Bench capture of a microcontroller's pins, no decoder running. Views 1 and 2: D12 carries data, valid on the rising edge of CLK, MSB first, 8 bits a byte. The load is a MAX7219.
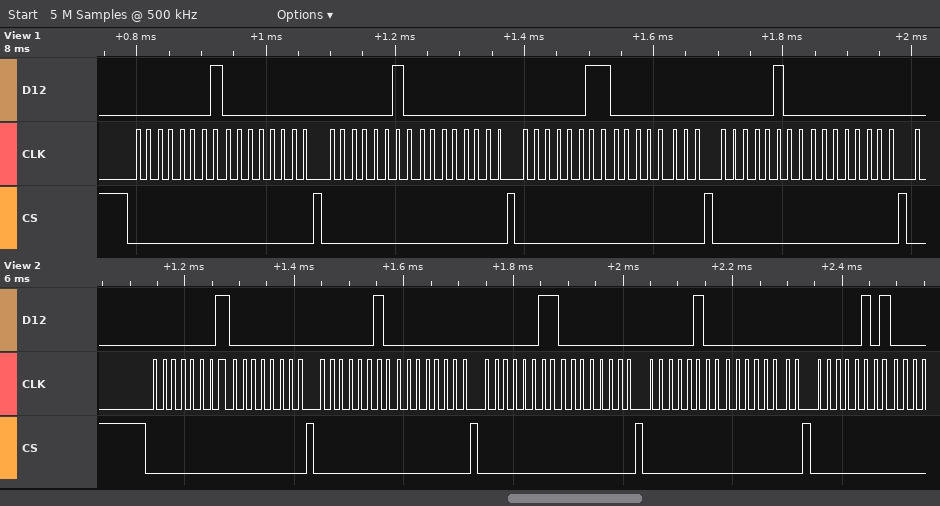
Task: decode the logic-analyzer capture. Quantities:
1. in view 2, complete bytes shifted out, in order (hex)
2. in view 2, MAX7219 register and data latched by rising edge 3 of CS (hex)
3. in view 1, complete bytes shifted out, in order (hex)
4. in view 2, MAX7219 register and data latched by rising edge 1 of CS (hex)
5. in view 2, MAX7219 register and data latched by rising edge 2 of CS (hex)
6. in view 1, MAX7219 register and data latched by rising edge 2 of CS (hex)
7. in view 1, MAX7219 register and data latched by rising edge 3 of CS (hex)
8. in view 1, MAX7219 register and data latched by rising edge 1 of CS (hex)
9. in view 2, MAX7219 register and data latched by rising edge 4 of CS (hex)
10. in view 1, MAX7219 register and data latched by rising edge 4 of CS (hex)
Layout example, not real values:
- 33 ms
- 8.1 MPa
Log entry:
- 01 00 02 00 03 00 04 00 05
- register 0x3, data 0x00
- 01 00 02 00 03 00 04 00
- register 0x1, data 0x00
- register 0x2, data 0x00
- register 0x2, data 0x00
- register 0x3, data 0x00
- register 0x1, data 0x00
- register 0x4, data 0x00
- register 0x4, data 0x00
